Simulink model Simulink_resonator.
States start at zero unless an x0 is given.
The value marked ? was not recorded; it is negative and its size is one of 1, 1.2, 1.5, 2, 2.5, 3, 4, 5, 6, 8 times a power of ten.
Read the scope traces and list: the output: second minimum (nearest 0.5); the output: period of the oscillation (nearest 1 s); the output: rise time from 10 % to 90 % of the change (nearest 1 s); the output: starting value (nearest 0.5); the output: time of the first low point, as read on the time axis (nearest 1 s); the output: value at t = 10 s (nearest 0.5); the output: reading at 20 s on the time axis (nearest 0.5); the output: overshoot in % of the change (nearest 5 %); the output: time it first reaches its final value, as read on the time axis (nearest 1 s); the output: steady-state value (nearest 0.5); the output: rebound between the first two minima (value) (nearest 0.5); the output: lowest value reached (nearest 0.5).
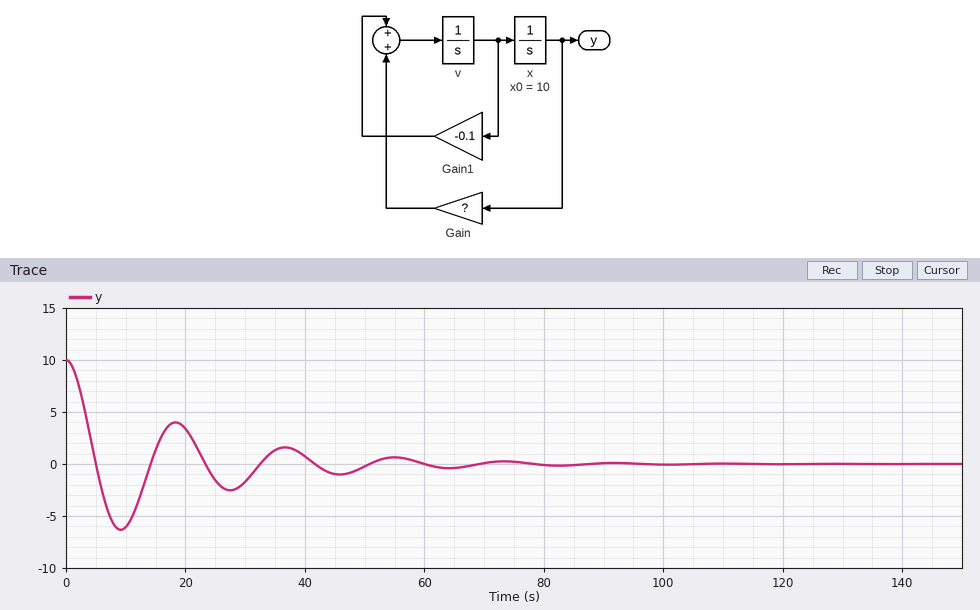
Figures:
-2.5
18 s
3 s
10.0
9 s
-6.0
3.5
65 %
5 s
0.0
4.0
-6.5
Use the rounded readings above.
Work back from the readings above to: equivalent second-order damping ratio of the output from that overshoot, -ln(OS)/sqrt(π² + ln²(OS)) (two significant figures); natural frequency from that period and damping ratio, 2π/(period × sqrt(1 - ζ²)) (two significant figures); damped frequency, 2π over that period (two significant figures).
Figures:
0.14
0.35 rad/s
0.35 rad/s
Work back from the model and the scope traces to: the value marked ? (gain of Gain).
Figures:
-0.12
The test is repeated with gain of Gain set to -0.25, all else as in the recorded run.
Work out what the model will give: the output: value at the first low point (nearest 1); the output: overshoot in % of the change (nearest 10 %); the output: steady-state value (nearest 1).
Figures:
-7
70 %
0
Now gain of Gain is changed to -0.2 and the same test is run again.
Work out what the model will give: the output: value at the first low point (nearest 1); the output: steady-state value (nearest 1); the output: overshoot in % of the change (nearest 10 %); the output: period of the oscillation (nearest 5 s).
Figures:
-7
0
70 %
15 s
